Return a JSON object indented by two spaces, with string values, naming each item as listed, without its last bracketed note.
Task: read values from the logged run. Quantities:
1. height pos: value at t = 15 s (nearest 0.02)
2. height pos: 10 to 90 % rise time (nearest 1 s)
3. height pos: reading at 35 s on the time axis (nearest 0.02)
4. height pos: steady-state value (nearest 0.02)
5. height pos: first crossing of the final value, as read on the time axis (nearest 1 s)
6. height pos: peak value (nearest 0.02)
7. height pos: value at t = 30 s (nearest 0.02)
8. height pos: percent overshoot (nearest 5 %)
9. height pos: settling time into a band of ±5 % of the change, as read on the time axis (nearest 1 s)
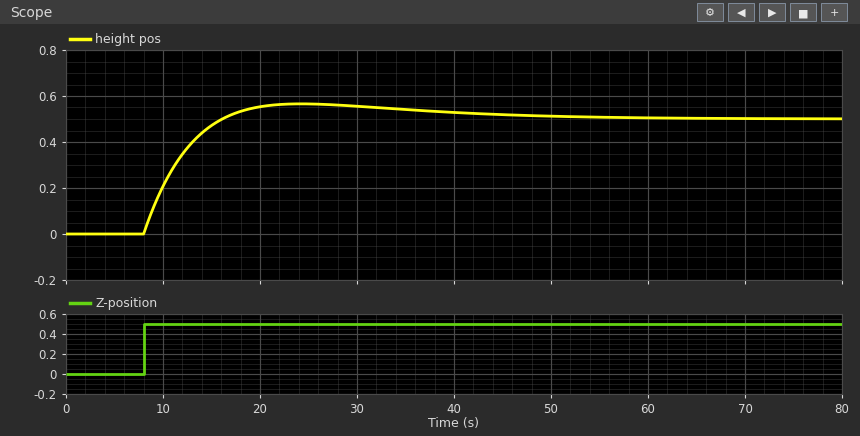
{
  "height pos: value at t = 15 s": "0.48",
  "height pos: 10 to 90 % rise time": "6 s",
  "height pos: reading at 35 s on the time axis": "0.54",
  "height pos: steady-state value": "0.50",
  "height pos: first crossing of the final value, as read on the time axis": "16 s",
  "height pos: peak value": "0.56",
  "height pos: value at t = 30 s": "0.56",
  "height pos: percent overshoot": "15 %",
  "height pos: settling time into a band of ±5 % of the change, as read on the time axis": "42 s"
}
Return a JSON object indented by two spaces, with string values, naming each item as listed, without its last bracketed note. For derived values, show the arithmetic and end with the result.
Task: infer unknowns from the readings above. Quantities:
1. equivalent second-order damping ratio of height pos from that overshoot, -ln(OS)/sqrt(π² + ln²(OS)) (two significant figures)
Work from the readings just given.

{
  "equivalent second-order damping ratio of height pos from that overshoot, -ln(OS)/sqrt(π² + ln²(OS))": "ln(0.15) = -1.897; 1.897 / sqrt(9.870 + 3.599) = 0.52"
}
